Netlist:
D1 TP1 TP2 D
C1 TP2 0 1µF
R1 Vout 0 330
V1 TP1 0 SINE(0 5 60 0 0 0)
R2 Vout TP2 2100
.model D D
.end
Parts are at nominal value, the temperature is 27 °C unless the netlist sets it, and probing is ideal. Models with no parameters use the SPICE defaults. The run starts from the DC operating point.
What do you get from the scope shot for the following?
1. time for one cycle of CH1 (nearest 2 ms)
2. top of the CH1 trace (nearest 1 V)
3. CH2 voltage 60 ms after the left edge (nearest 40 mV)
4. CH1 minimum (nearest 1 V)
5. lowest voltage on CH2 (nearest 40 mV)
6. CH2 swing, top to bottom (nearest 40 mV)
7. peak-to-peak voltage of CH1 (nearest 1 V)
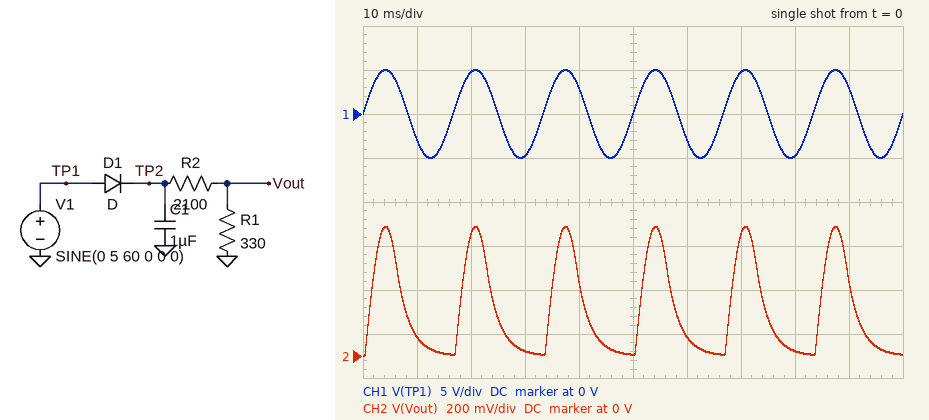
16 ms
5 V
80 mV
-5 V
0 V
600 mV
10 V
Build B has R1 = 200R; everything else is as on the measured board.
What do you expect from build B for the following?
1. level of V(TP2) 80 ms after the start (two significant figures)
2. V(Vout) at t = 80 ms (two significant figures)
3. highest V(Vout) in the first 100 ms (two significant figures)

140 mV
12 mV
380 mV
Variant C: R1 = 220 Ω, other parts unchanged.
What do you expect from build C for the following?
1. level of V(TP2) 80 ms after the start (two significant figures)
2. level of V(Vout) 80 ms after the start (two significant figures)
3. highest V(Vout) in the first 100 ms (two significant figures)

140 mV
13 mV
410 mV
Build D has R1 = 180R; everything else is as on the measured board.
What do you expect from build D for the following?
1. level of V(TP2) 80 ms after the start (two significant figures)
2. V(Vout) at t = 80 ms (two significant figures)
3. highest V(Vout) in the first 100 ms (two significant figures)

130 mV
10 mV
340 mV
